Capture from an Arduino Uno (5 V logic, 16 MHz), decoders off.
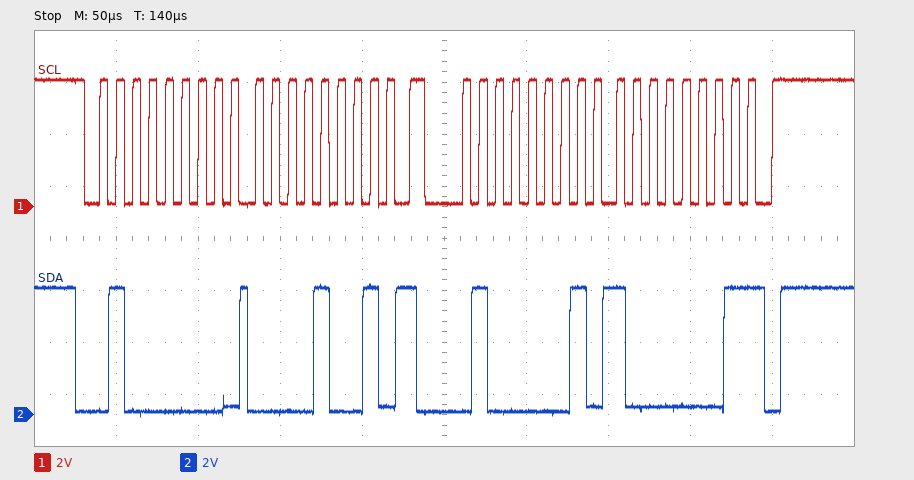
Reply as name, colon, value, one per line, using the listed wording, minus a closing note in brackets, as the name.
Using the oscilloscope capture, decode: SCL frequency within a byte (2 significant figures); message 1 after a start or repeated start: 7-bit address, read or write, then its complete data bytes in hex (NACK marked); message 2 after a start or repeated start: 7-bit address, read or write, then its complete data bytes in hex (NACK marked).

SCL frequency within a byte: 100 kHz
message 1 after a start or repeated start: 7-bit address, read or write, then its complete data bytes in hex: 0x20 write: 09
message 2 after a start or repeated start: 7-bit address, read or write, then its complete data bytes in hex: 0x20 read: 81 NACK
